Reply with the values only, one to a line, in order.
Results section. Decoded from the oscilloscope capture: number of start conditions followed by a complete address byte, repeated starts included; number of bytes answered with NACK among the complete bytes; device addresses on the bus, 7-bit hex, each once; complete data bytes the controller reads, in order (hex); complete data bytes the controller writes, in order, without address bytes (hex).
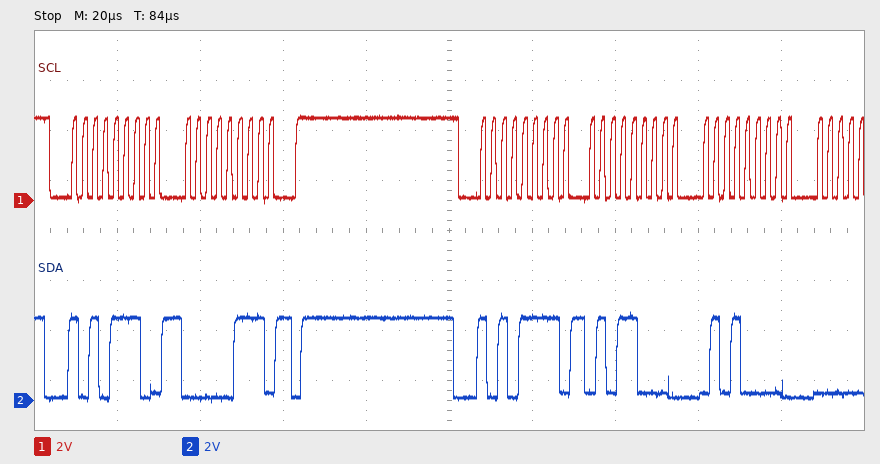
2
0
0x57
58 50
07
